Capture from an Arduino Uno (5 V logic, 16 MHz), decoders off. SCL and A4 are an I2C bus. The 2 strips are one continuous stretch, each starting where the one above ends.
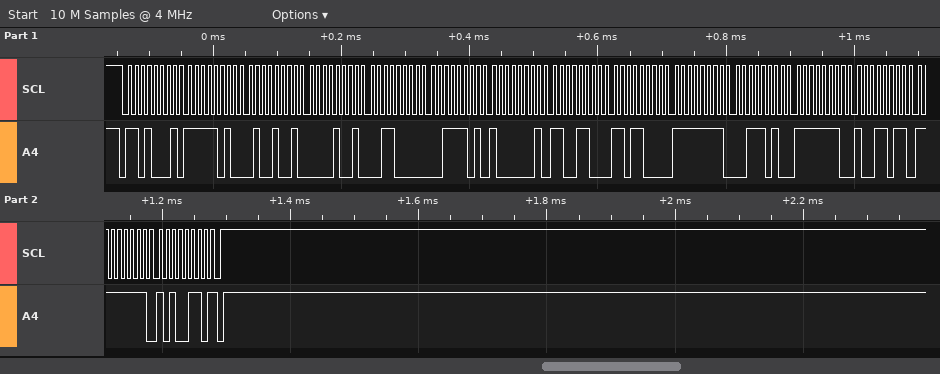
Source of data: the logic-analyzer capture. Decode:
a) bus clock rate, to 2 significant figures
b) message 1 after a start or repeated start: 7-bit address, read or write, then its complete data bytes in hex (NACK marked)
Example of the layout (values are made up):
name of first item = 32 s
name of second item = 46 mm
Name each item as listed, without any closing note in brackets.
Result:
bus clock rate, to 2 significant figures = 100 kHz
message 1 after a start or repeated start: 7-bit address, read or write, then its complete data bytes in hex = 0x68 read: FA 49 09 30 3D 81 CC D8 FF 3A FE 9B FF A6 NACK
